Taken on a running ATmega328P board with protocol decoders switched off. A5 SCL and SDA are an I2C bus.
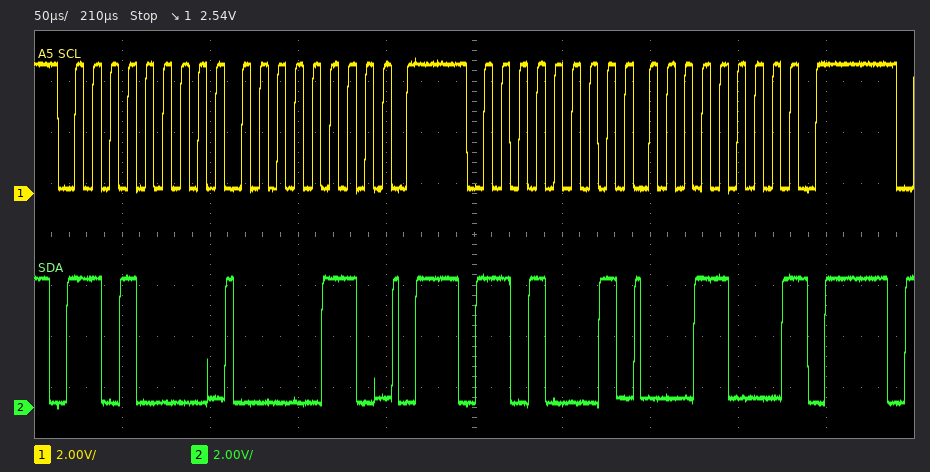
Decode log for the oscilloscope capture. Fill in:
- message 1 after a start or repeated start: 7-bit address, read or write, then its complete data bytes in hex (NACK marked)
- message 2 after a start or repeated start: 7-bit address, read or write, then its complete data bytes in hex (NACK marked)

0x68 write: 06
0x68 read: 18 NACK
